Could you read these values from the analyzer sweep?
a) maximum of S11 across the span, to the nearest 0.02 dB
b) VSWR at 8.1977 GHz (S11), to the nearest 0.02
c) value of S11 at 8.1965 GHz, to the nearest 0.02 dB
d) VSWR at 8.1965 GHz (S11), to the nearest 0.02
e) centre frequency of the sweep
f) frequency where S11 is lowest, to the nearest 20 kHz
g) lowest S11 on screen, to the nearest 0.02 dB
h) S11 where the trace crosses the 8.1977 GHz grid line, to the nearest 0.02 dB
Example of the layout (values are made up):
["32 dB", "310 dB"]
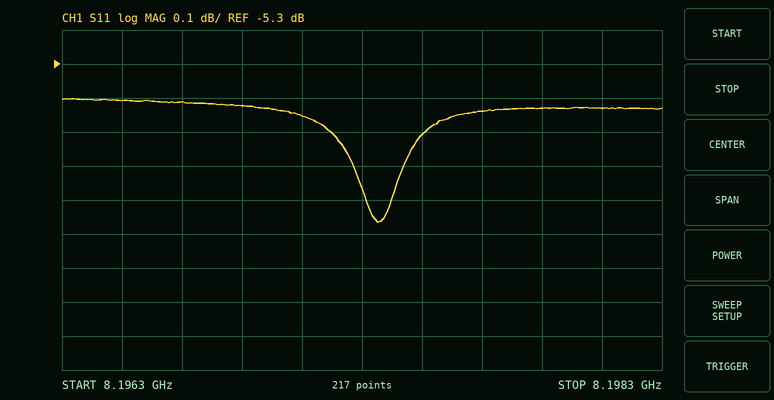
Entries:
["-5.40 dB", "3.30", "-5.40 dB", "3.32", "8.1973 GHz", "8.19736 GHz", "-5.76 dB", "-5.44 dB"]
